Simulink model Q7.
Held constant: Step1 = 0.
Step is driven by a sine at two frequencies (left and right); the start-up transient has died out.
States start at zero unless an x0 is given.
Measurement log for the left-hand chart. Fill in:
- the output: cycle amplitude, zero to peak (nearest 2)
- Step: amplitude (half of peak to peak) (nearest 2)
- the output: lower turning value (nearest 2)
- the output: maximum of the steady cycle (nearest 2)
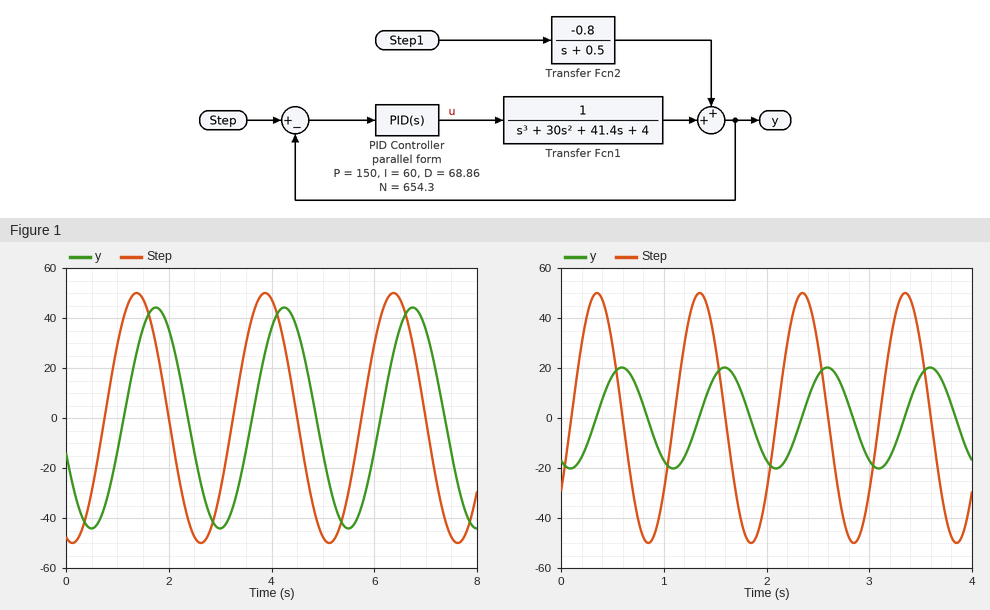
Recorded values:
44
50
-44
44
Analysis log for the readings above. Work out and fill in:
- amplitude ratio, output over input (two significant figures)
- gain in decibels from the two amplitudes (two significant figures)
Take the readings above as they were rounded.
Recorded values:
0.88
-1.1 dB
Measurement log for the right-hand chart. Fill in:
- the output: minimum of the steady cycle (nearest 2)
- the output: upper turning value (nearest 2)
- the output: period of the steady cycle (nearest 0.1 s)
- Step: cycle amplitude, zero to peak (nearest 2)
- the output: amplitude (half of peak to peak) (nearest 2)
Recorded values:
-20
20
1.0 s
50
20
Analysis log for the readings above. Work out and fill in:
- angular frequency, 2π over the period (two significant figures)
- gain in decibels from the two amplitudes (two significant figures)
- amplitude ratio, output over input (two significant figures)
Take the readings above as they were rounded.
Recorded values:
6.3 rad/s
-8.0 dB
0.40
